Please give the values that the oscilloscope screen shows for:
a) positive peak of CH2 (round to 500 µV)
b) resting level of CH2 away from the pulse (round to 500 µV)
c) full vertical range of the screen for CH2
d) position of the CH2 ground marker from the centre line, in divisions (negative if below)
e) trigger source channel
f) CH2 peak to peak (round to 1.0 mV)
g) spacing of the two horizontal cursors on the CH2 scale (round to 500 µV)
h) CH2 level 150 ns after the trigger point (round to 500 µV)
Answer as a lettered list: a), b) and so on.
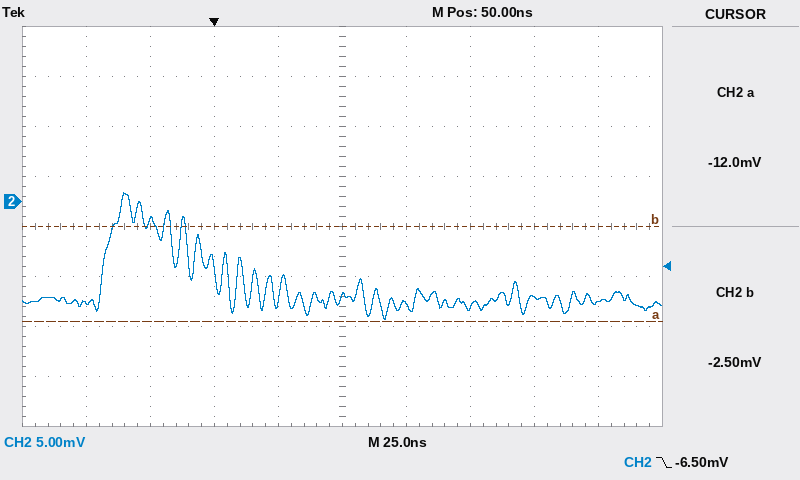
a) 1.0 mV
b) -10.0 mV
c) 40 mV
d) +0.5 div
e) CH2
f) 13.0 mV
g) 9.5 mV
h) -10.0 mV
